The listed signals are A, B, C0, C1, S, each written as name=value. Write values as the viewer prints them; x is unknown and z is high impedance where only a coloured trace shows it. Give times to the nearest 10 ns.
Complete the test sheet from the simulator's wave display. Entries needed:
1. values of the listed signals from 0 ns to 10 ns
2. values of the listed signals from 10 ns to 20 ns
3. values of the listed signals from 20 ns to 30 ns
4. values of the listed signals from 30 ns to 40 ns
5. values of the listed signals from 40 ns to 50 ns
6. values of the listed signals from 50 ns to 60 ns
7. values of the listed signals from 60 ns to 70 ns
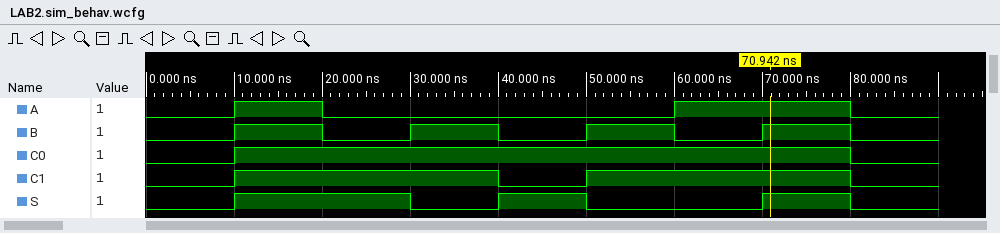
A=0, B=0, C0=0, C1=0, S=0
A=1, B=1, C0=1, C1=1, S=1
A=0, B=0, C0=1, C1=1, S=1
A=0, B=1, C0=1, C1=1, S=0
A=0, B=0, C0=1, C1=0, S=1
A=0, B=1, C0=1, C1=1, S=0
A=1, B=0, C0=1, C1=1, S=0
